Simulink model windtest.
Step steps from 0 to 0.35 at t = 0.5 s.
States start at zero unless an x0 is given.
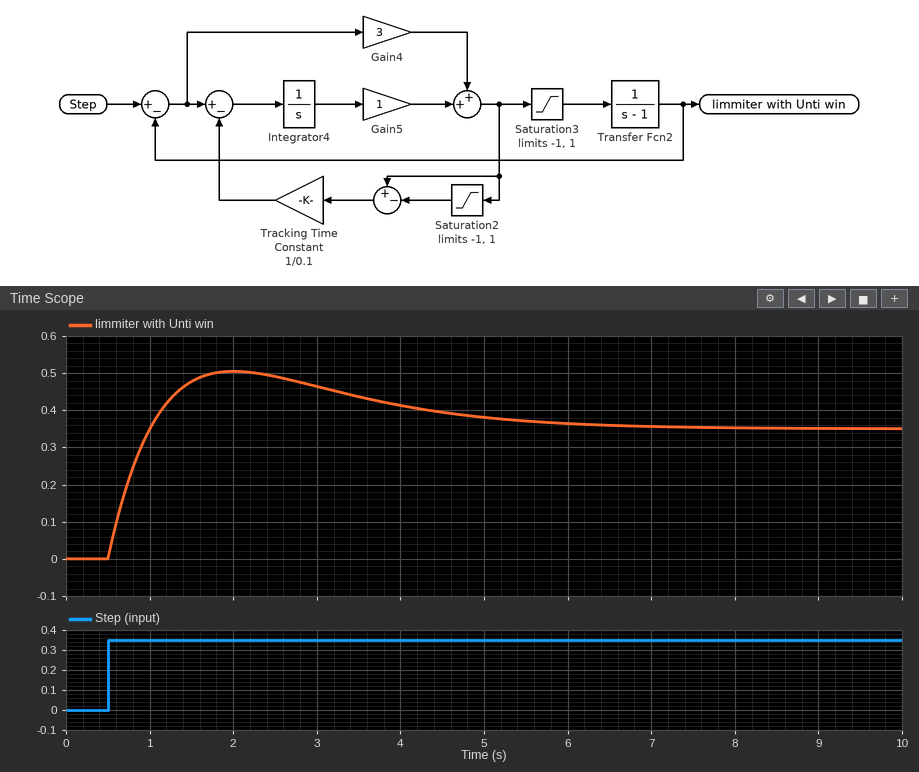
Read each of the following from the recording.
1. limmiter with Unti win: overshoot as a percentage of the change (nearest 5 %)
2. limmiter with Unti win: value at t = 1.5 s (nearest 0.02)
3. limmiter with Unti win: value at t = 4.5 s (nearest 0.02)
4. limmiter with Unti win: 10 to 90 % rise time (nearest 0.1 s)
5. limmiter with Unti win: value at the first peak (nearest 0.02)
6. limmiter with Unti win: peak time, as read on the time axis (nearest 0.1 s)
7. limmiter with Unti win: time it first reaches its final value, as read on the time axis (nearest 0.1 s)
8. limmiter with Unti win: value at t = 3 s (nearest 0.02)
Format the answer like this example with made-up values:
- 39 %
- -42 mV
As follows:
- 45 %
- 0.48
- 0.40
- 0.4 s
- 0.50
- 2.0 s
- 1.0 s
- 0.46
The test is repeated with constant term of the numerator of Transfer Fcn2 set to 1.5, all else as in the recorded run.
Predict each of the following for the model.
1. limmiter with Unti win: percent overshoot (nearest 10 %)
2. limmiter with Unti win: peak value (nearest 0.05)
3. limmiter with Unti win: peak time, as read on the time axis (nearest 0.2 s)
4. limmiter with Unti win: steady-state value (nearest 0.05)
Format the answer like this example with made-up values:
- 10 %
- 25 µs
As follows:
- 30 %
- 0.45
- 1.6 s
- 0.35
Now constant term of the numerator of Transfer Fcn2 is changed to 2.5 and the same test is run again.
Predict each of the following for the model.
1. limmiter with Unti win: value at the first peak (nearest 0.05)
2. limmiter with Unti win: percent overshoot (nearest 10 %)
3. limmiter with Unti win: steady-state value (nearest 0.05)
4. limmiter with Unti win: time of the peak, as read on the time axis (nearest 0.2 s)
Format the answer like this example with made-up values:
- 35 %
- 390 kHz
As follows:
- 0.40
- 20 %
- 0.35
- 1.2 s
